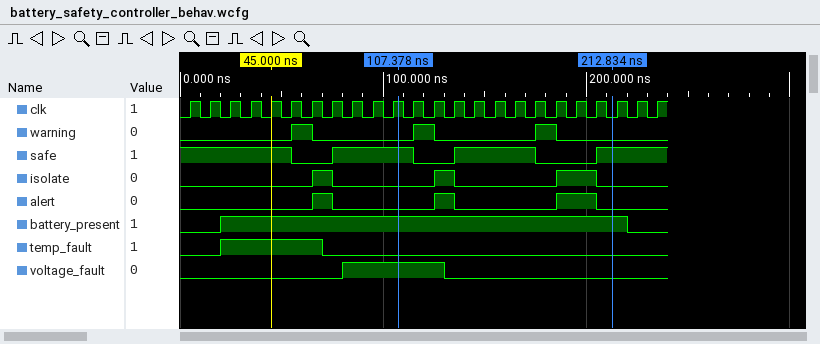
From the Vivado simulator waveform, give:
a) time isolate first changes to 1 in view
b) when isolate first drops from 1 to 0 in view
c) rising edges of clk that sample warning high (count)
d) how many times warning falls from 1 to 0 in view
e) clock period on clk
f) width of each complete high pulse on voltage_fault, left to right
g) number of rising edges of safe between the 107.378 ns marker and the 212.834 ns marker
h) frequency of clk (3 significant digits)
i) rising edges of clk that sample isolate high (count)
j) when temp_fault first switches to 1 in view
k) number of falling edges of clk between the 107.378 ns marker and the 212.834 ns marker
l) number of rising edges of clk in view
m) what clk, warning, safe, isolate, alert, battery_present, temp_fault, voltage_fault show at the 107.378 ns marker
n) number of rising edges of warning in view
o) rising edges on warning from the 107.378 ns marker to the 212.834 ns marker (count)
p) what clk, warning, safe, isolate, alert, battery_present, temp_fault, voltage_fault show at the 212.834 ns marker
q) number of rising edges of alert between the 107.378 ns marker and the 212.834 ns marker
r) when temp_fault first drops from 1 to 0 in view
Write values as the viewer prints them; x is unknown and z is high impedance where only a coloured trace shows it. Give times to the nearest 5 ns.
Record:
65 ns
75 ns
3
3
10 ns
50 ns
2
100 MHz
4
20 ns
11
24
clk=1, warning=0, safe=1, isolate=0, alert=0, battery_present=1, temp_fault=0, voltage_fault=1
3
2
clk=0, warning=0, safe=1, isolate=0, alert=0, battery_present=1, temp_fault=0, voltage_fault=0
2
70 ns
